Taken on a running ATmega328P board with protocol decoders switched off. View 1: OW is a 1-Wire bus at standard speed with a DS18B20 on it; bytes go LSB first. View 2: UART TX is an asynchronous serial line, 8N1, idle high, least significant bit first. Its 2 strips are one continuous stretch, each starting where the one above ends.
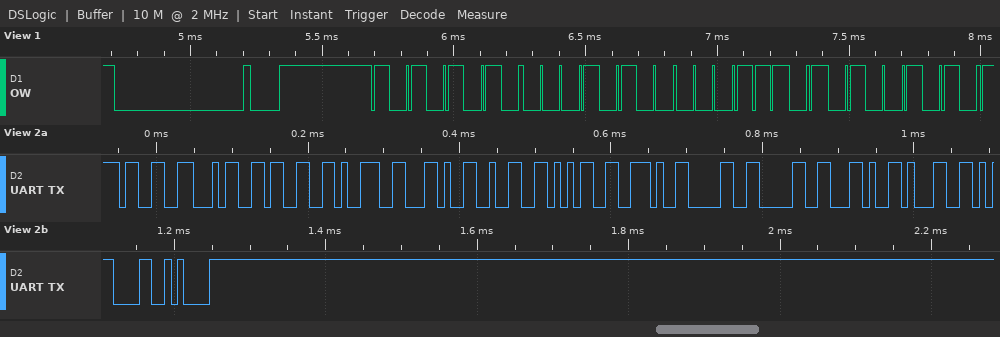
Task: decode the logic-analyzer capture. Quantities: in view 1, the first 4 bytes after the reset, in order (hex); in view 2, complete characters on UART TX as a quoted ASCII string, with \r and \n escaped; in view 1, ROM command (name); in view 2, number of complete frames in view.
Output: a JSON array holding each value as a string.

["55 28 B8 52", "\"3439,25.00,1\\r\\n\"", "Match ROM", "14"]
